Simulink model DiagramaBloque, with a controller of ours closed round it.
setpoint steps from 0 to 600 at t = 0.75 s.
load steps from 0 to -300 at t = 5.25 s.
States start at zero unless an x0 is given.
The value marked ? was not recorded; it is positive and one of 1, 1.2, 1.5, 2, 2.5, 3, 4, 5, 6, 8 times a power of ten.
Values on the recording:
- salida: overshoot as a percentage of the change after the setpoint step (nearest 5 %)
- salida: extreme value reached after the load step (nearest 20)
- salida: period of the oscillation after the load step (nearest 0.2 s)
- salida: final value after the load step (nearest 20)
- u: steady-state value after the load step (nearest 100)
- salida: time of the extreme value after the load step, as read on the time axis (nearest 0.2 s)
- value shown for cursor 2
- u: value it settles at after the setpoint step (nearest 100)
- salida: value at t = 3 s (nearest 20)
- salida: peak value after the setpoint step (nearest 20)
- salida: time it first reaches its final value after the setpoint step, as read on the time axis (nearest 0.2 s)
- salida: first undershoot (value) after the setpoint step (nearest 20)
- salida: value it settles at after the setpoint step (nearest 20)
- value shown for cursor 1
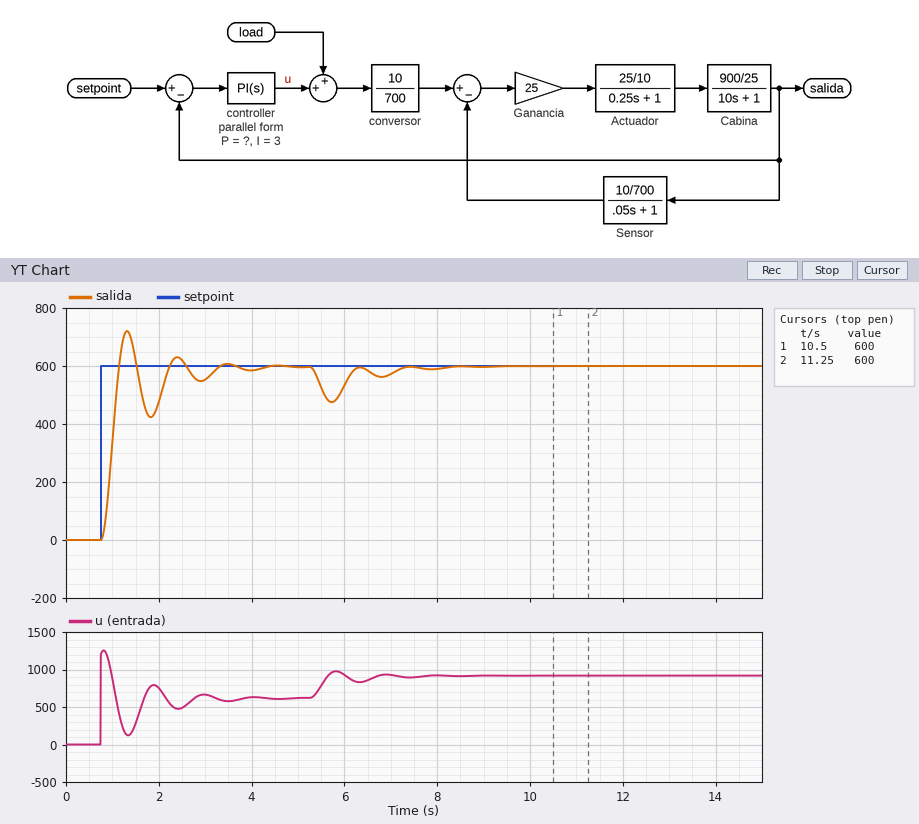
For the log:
20 %
480
1.0 s
600
900
5.8 s
600
600
560
720
1.2 s
420
600
600
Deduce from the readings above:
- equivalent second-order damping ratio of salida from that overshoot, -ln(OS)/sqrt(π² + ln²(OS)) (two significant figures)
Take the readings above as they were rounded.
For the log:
0.46
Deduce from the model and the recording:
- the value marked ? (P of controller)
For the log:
2
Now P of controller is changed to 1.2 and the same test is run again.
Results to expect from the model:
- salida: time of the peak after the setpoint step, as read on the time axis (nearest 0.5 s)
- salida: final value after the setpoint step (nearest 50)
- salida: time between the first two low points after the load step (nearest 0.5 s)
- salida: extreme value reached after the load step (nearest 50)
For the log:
1.5 s
600
1.5 s
450
